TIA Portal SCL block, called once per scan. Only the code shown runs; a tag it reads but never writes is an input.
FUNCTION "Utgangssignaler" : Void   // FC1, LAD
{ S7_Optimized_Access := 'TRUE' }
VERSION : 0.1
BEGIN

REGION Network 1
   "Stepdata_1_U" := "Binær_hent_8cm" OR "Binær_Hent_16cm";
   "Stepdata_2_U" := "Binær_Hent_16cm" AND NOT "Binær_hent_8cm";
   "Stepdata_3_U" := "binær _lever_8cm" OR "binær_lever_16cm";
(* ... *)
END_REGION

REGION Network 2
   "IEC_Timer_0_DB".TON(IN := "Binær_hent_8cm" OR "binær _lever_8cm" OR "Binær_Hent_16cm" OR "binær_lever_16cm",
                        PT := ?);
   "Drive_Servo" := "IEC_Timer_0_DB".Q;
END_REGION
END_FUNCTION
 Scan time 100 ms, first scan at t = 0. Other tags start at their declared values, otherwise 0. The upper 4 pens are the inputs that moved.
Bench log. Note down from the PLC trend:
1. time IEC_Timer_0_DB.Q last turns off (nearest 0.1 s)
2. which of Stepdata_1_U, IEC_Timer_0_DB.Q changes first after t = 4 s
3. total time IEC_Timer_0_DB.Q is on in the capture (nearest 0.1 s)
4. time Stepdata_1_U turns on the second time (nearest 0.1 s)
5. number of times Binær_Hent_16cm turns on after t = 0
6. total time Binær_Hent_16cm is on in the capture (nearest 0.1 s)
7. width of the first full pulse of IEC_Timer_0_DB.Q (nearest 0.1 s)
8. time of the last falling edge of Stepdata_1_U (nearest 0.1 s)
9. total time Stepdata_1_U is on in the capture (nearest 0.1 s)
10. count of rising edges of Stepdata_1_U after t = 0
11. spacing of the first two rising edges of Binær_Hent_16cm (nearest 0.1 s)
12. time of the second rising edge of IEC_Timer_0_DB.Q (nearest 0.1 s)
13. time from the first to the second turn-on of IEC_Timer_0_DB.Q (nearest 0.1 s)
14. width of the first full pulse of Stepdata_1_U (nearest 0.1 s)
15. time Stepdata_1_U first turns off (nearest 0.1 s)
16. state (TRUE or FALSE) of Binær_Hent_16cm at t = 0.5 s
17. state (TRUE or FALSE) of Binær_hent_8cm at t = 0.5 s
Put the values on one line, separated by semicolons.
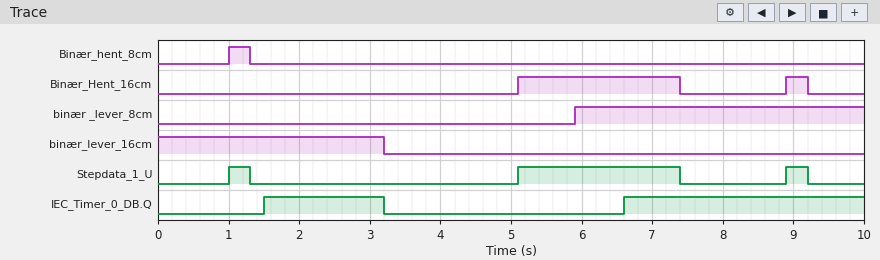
3.2 s; Stepdata_1_U; 5.1 s; 5.1 s; 2; 2.6 s; 1.7 s; 9.2 s; 2.9 s; 3; 3.8 s; 6.6 s; 5.1 s; 0.3 s; 1.3 s; FALSE; FALSE
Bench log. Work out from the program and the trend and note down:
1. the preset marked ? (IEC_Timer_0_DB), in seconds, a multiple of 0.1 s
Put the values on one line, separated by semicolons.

1.5 s
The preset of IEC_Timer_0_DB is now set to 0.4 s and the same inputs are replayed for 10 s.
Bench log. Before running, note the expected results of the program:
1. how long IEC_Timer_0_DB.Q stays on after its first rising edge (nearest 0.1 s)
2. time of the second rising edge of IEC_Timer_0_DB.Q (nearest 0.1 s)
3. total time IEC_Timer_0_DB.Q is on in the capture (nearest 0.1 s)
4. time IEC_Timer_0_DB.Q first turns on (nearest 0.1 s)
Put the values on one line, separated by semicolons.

2.8 s; 5.5 s; 7.3 s; 0.4 s
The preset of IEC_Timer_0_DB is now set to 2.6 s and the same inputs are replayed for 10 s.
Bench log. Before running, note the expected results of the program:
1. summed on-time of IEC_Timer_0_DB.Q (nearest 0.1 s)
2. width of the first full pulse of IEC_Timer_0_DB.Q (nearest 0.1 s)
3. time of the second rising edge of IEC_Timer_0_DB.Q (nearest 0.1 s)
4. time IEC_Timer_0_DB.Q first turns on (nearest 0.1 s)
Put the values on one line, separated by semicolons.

2.9 s; 0.6 s; 7.7 s; 2.6 s
